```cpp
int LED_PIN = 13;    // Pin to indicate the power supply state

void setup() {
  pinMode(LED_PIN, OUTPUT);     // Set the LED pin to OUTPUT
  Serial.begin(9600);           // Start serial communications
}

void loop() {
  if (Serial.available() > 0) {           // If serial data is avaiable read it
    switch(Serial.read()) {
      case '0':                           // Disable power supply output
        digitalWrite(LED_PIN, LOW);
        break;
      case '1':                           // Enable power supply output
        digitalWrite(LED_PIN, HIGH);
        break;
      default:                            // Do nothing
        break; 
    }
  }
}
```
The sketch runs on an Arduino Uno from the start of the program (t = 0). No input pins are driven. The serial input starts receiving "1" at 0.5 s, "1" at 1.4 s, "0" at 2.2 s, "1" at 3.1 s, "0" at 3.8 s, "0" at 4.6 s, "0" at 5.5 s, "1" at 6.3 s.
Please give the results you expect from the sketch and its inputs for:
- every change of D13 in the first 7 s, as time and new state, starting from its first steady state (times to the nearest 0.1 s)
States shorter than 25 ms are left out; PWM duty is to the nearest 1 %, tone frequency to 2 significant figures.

0 s low; 0.5 s high; 2.2 s low; 3.1 s high; 3.8 s low; 6.3 s high
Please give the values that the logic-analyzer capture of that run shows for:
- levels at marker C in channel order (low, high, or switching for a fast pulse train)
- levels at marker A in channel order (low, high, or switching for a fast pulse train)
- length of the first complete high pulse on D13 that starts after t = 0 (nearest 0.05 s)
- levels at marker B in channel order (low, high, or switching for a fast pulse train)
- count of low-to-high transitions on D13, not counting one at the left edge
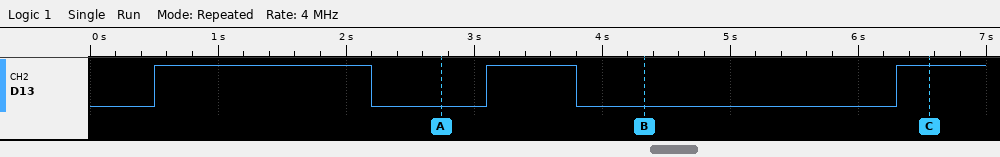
D13 high
D13 low
1.70 s
D13 low
3
